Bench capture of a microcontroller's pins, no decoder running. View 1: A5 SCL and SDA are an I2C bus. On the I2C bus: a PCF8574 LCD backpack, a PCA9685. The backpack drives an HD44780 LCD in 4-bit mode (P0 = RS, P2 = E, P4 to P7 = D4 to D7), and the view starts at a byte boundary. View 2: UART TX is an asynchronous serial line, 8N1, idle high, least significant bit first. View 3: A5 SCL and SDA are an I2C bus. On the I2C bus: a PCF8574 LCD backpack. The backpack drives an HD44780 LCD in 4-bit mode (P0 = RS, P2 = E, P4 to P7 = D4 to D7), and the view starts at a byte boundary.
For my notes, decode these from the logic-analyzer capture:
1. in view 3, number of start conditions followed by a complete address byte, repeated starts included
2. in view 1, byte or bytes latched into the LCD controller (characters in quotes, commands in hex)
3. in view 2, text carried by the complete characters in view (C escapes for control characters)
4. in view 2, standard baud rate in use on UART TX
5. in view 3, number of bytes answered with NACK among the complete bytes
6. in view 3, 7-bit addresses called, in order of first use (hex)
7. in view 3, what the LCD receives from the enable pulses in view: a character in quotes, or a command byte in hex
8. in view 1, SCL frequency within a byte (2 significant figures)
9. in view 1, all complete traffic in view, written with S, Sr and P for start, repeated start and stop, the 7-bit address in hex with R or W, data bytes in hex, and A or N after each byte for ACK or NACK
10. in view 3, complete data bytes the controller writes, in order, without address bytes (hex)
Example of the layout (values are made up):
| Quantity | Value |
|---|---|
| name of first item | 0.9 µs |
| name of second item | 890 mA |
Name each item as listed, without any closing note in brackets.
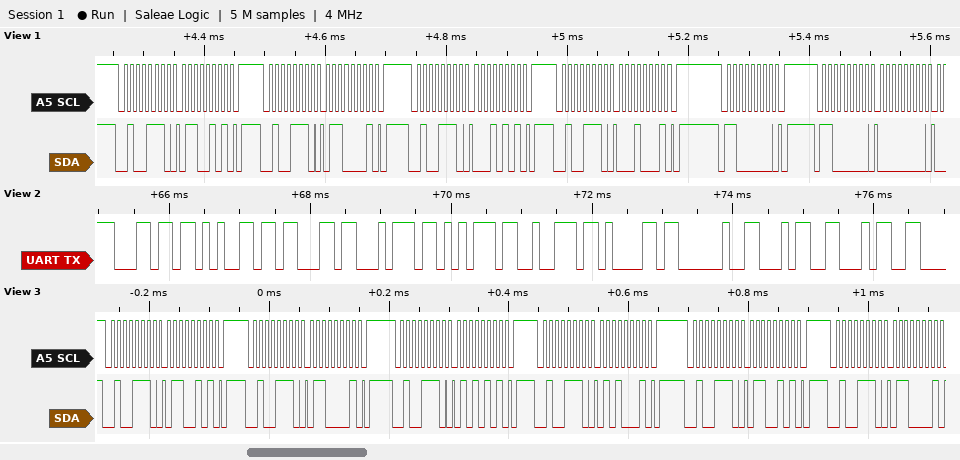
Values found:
| Quantity | Value |
|---|---|
| in view 3, number of start conditions followed by a complete address byte, repeated starts included | 6 |
| in view 1, byte or bytes latched into the LCD controller | 'a' |
| in view 2, text carried by the complete characters in view | "lectura 44" |
| in view 2, standard baud rate in use on UART TX | 9600 baud |
| in view 3, number of bytes answered with NACK among the complete bytes | 0 |
| in view 3, 7-bit addresses called, in order of first use | 0x27 |
| in view 3, what the LCD receives from the enable pulses in view: a character in quotes, or a command byte in hex | 'e' |
| in view 1, SCL frequency within a byte | 100 kHz |
| in view 1, all complete traffic in view, written with S, Sr and P for start, repeated start and stop, the 7-bit address in hex with R or W, data bytes in hex, and A or N after each byte for ACK or NACK | S 27W A 65 A P S 27W A 61 A P S 27W A 15 A P S 27W A 11 A P S 60W A P S 60W A 00 A |
| in view 3, complete data bytes the controller writes, in order, without address bytes | 65 61 55 51 65 61 |
